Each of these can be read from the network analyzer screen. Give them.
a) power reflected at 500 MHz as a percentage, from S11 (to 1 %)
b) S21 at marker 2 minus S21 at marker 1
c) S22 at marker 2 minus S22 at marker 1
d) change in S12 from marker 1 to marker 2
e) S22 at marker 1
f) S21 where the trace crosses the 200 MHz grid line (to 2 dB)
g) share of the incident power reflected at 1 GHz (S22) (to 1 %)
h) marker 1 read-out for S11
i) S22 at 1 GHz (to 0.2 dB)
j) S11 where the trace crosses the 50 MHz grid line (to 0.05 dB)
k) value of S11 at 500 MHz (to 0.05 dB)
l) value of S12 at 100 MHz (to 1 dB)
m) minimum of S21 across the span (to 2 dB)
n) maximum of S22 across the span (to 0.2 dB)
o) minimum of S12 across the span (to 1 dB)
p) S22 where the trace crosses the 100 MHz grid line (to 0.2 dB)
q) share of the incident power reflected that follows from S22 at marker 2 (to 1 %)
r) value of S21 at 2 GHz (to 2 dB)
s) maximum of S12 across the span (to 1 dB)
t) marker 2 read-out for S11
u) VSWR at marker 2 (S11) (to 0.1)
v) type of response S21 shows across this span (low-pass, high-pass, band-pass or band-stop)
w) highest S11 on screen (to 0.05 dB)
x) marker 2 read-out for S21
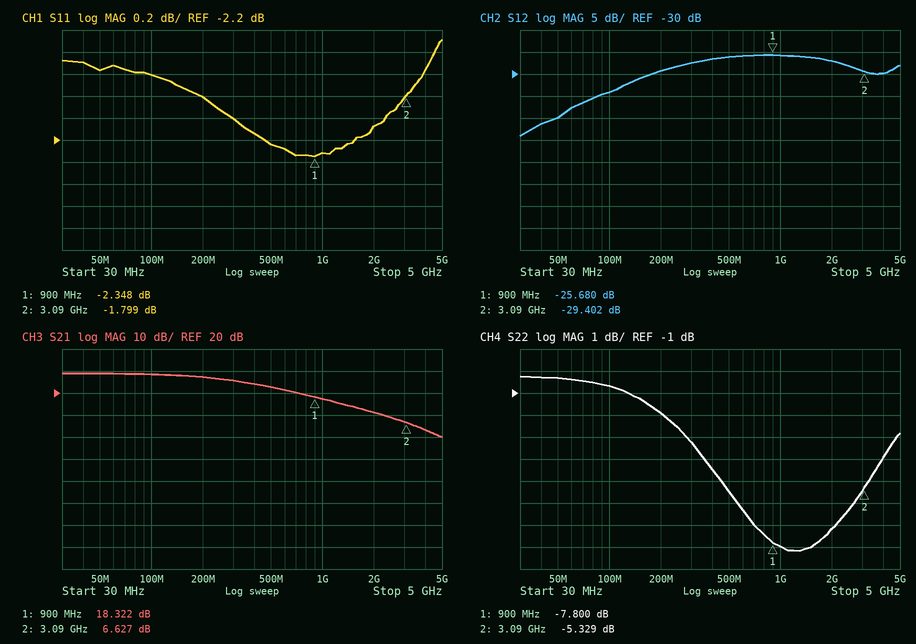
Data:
60 %
-11.695 dB
2.471 dB
-3.722 dB
-7.800 dB
28 dB
16 %
-2.348 dB
-8.0 dB
-1.55 dB
-2.25 dB
-34 dB
0 dB
-0.2 dB
-44 dB
-0.6 dB
29 %
12 dB
-26 dB
-1.799 dB
9.7
low-pass
-1.30 dB
6.627 dB
